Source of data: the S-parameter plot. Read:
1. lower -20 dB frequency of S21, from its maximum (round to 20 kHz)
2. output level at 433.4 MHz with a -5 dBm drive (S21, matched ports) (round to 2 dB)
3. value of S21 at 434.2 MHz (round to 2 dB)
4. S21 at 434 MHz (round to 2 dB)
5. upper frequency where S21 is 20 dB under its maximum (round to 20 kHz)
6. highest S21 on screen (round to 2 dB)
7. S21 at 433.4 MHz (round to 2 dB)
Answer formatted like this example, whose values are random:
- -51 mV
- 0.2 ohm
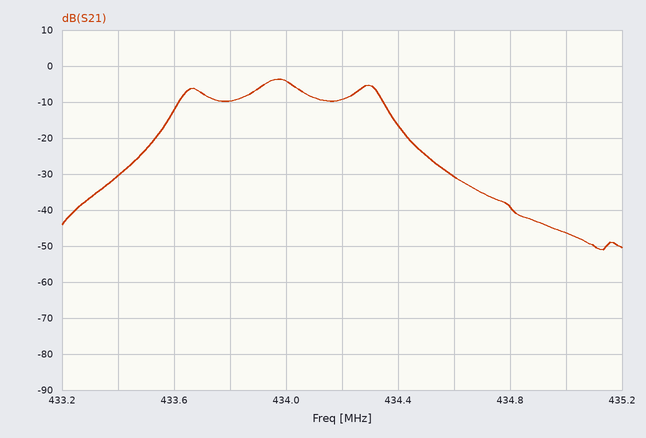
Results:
- 433.50 MHz
- -36 dBm
- -10 dB
- -4 dB
- 434.48 MHz
- -4 dB
- -30 dB
